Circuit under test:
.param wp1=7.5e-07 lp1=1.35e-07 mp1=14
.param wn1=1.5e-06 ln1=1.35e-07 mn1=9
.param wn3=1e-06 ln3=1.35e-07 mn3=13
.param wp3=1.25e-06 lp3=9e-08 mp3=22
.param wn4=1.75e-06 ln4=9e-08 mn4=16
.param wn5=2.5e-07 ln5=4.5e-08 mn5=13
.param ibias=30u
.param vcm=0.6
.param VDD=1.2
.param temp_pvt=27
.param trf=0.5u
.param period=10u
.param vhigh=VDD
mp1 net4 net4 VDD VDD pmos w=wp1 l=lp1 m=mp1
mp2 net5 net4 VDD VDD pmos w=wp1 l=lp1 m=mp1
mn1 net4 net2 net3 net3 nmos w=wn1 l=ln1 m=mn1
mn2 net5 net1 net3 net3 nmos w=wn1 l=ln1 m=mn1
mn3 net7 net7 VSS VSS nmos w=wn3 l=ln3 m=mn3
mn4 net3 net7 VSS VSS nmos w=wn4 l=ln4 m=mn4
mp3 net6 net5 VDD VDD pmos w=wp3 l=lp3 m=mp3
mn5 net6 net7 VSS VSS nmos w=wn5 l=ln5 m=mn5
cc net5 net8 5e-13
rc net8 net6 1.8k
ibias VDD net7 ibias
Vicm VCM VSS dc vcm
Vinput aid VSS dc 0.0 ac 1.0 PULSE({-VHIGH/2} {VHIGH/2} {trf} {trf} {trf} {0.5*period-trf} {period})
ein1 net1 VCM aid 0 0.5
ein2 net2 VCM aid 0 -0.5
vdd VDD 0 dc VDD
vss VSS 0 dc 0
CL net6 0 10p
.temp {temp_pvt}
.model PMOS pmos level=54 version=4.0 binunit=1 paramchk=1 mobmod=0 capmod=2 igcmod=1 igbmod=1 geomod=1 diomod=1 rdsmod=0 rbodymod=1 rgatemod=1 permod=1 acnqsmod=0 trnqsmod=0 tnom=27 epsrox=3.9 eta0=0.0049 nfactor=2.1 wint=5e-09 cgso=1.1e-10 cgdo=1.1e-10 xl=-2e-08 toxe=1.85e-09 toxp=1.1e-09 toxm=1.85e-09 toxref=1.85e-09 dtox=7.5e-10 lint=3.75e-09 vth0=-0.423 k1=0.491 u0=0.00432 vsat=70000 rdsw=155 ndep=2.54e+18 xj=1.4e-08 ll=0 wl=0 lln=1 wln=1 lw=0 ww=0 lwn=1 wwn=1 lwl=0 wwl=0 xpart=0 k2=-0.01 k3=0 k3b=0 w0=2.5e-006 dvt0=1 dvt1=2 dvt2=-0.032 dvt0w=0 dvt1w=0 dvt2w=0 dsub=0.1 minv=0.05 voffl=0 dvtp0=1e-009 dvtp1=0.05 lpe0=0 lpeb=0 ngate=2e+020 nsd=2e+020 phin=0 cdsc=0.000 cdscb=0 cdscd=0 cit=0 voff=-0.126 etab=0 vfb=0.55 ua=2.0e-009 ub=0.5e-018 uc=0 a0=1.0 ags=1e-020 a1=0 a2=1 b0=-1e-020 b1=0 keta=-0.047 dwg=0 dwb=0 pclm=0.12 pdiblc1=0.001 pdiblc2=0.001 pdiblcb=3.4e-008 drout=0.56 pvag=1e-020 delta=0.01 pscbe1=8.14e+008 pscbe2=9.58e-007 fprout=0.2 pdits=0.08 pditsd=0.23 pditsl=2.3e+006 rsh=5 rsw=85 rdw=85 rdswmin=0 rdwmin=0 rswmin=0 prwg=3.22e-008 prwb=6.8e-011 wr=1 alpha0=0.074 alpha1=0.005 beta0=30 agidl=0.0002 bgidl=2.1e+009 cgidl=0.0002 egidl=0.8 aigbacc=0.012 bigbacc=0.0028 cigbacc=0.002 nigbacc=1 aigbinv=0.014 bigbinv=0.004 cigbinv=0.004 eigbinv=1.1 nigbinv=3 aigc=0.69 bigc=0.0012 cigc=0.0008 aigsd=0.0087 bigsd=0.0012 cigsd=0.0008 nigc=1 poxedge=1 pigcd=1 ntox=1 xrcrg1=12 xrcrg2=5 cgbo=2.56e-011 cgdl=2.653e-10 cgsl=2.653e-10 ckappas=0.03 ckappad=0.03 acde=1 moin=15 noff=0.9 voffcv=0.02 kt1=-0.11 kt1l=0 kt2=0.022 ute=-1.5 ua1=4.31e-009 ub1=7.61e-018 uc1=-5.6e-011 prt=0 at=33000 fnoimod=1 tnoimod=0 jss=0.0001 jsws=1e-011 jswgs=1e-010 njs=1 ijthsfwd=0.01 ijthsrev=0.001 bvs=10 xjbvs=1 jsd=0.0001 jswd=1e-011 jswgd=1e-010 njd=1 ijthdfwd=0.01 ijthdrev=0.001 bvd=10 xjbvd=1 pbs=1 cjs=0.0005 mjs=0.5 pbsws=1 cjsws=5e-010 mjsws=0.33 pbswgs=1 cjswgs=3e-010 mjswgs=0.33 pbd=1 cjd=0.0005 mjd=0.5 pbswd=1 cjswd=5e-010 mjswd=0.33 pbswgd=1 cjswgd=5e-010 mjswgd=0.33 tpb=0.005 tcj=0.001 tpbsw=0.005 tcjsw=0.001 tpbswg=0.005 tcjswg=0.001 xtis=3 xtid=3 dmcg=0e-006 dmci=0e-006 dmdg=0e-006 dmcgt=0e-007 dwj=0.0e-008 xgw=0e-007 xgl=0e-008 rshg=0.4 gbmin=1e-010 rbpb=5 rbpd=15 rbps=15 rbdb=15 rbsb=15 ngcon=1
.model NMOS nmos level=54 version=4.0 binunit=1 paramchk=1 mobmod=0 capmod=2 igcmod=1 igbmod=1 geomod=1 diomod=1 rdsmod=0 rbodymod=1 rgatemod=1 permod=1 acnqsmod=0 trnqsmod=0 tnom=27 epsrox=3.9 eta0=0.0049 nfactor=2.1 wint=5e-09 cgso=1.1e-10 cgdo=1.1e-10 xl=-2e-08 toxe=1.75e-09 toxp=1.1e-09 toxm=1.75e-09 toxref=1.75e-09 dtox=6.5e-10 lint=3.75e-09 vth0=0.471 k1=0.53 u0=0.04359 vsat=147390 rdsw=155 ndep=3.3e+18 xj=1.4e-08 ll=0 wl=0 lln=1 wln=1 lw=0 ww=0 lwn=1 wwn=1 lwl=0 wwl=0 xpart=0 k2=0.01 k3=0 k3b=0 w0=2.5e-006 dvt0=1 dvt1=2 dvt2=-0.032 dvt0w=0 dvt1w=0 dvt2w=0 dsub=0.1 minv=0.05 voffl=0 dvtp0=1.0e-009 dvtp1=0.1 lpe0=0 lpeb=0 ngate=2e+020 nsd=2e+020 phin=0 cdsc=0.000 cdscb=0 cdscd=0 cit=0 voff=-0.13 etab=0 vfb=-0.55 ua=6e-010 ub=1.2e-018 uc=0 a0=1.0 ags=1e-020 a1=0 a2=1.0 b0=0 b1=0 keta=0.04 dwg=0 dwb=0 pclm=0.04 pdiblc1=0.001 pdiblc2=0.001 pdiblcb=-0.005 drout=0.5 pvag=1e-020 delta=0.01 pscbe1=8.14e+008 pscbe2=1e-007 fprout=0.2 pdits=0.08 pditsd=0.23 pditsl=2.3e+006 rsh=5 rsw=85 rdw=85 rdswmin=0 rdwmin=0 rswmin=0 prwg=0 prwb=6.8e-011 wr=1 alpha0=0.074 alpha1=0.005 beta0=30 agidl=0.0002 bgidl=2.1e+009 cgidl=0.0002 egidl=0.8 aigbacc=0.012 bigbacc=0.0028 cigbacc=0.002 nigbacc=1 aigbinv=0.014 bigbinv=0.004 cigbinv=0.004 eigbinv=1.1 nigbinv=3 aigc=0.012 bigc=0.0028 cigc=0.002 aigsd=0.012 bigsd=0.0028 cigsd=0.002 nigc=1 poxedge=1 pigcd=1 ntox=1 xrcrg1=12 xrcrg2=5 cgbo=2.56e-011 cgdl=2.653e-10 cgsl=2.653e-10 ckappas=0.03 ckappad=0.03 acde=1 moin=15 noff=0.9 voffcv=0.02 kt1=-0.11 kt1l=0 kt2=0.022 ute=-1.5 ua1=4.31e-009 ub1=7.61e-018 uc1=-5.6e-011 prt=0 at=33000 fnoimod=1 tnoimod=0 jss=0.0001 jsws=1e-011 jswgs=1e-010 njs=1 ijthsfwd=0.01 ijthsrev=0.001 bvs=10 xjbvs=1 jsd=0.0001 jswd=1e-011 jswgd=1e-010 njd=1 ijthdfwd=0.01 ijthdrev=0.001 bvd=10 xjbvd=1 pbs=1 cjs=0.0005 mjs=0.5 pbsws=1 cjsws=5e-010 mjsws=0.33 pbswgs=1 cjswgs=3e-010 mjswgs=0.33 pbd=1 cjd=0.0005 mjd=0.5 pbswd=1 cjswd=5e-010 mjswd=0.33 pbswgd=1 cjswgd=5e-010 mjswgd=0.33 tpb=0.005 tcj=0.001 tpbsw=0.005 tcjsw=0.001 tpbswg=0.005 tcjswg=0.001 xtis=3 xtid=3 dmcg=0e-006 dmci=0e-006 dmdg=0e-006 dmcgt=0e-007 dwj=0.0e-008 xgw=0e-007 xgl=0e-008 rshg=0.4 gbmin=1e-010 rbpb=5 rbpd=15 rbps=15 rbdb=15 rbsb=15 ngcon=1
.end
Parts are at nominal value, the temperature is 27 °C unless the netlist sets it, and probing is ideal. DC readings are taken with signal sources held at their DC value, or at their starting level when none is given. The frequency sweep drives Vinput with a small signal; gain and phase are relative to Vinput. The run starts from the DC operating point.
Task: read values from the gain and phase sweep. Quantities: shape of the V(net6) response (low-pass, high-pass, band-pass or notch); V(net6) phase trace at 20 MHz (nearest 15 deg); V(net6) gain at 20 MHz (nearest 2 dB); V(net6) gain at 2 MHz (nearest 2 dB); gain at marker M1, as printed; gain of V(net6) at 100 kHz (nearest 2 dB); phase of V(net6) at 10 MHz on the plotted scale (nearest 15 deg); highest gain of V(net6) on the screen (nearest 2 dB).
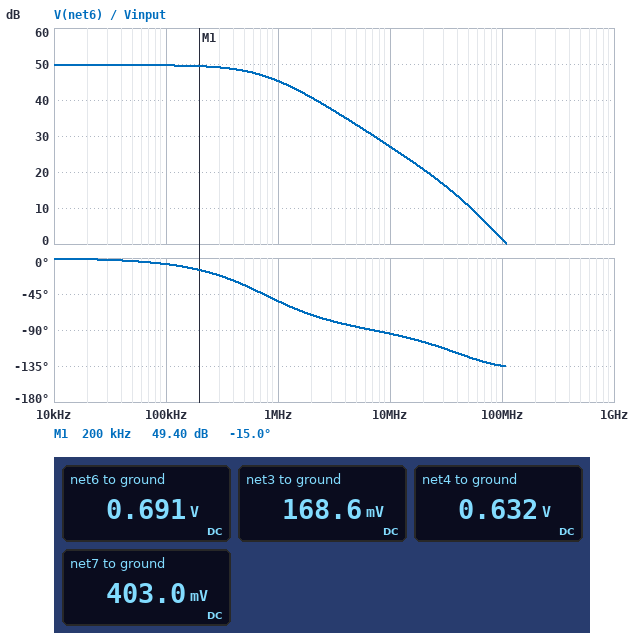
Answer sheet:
low-pass
-105 deg
20 dB
40 dB
49.40 dB
50 dB
-90 deg
50 dB
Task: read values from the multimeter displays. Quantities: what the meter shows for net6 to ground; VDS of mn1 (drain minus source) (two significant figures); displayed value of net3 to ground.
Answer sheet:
0.691 V
460 mV
168.6 mV
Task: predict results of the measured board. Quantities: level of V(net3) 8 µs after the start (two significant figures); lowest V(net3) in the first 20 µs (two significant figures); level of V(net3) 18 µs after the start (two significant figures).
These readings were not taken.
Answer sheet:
420 mV
2.6 mV
420 mV
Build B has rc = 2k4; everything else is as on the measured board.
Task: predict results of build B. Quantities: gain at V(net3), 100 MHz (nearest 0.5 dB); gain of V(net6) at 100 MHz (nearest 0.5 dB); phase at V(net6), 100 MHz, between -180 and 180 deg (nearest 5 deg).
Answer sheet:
-38.5 dB
2.0 dB
-130 deg
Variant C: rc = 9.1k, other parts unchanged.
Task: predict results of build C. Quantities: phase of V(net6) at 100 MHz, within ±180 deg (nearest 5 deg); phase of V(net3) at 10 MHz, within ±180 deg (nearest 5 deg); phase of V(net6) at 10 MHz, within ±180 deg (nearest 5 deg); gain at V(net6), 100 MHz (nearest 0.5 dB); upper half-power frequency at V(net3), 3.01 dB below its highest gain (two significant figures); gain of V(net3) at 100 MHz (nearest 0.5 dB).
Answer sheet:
-105 deg
145 deg
-85 deg
9.5 dB
750 kHz
-30.5 dB
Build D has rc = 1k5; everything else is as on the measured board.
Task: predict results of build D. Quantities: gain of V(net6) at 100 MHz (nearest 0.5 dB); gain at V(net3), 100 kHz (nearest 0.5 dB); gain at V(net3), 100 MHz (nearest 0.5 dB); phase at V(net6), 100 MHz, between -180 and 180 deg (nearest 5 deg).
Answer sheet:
1.0 dB
-11.5 dB
-39.5 dB
-140 deg
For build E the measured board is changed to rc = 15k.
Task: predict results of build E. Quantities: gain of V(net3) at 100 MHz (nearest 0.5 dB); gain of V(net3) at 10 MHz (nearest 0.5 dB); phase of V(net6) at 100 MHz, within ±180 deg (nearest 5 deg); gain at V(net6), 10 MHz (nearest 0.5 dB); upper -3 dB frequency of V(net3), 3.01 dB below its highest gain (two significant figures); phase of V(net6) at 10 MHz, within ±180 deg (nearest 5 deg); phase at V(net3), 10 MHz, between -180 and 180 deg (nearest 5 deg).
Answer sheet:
-27.0 dB
-30.5 dB
-110 deg
27.5 dB
740 kHz
-75 deg
155 deg
